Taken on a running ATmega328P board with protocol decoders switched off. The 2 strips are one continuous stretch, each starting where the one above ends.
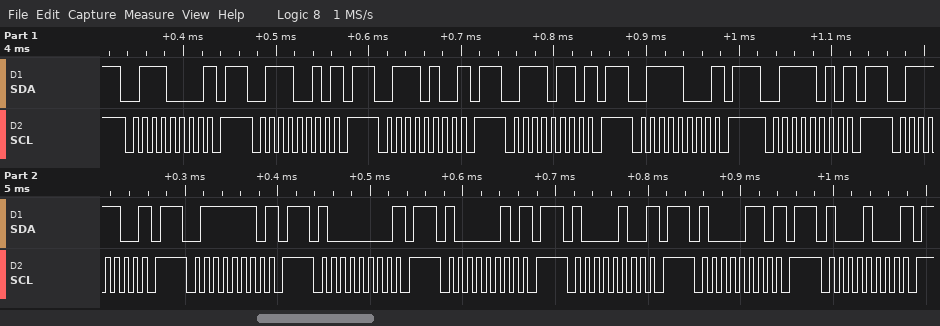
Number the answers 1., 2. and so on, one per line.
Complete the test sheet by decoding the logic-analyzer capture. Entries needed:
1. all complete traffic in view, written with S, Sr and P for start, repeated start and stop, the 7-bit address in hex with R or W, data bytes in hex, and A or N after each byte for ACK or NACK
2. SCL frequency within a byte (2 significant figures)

1. S 38W N P S 39W N P S 3AW N P S 3BW N P S 3CW N P S 3DW N P S 3EW N P S 3FW N P S 40W N P S 41W N P S 42W N P S 43W N P S 44W N P
2. 100 kHz
